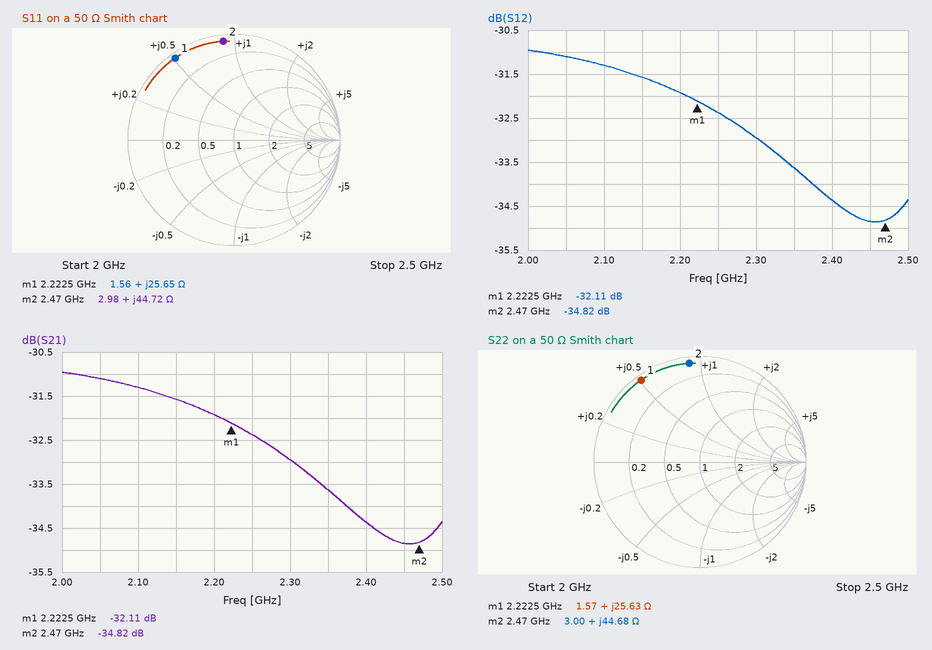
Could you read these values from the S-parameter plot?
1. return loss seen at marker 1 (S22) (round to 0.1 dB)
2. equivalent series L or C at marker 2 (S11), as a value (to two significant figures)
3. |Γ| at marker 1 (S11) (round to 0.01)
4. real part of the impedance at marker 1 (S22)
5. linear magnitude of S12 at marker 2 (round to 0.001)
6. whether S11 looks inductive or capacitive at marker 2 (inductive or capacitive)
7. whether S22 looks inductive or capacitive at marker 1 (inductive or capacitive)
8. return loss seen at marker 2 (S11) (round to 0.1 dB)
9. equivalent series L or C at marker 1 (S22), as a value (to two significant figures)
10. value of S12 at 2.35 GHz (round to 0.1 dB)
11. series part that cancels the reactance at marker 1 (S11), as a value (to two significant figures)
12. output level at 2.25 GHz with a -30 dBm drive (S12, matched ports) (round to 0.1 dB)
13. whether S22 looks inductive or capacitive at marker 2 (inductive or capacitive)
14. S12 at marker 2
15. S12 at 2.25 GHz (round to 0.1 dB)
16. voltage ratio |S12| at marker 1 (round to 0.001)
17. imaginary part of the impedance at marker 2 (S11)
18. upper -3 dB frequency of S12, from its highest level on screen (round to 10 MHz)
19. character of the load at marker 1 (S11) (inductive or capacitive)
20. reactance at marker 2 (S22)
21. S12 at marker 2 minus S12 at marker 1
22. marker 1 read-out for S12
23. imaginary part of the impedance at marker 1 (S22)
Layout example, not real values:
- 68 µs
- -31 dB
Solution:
- 0.4 dB
- 2.9 nH
- 0.95
- 1.57 Ω
- 0.018
- inductive
- inductive
- 0.6 dB
- 1.8 nH
- -33.6 dB
- 2.8 pF
- -62.4 dBm
- inductive
- -34.82 dB
- -32.4 dB
- 0.025
- +44.72 Ω
- 2.37 GHz
- inductive
- +44.68 Ω
- -2.71 dB
- -32.11 dB
- +25.63 Ω
